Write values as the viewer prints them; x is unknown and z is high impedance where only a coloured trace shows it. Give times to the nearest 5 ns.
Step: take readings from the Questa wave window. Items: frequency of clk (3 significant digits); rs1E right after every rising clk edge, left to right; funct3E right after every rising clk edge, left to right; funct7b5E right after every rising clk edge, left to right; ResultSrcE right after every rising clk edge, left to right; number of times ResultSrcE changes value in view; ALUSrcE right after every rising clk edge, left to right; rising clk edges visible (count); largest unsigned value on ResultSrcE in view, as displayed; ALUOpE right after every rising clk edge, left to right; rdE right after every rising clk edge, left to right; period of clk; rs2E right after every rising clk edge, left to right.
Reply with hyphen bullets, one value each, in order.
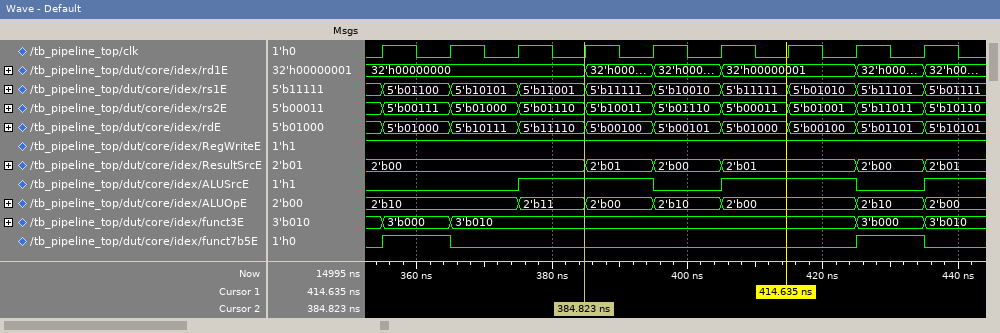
- 100 MHz
- 5'b01100, 5'b10101, 5'b11001, 5'b11111, 5'b10010, 5'b11111, 5'b01010, 5'b11101, 5'b01111
- 3'b000, 3'b010, 3'b010, 3'b010, 3'b010, 3'b010, 3'b010, 3'b000, 3'b010
- 1 0 0 0 0 0 0 1 0
- 2'b00, 2'b00, 2'b00, 2'b01, 2'b00, 2'b01, 2'b01, 2'b00, 2'b01
- 5
- 0 0 1 1 0 1 1 0 1
- 9
- 2'b01
- 2'b10, 2'b10, 2'b11, 2'b00, 2'b10, 2'b00, 2'b00, 2'b10, 2'b00
- 5'b01000, 5'b10111, 5'b11110, 5'b00100, 5'b00101, 5'b01000, 5'b00100, 5'b01101, 5'b10101
- 10 ns
- 5'b00111, 5'b01000, 5'b01110, 5'b10011, 5'b01110, 5'b00011, 5'b01001, 5'b11011, 5'b10110
